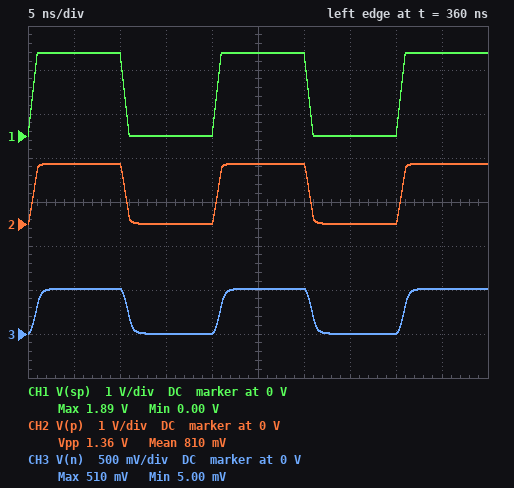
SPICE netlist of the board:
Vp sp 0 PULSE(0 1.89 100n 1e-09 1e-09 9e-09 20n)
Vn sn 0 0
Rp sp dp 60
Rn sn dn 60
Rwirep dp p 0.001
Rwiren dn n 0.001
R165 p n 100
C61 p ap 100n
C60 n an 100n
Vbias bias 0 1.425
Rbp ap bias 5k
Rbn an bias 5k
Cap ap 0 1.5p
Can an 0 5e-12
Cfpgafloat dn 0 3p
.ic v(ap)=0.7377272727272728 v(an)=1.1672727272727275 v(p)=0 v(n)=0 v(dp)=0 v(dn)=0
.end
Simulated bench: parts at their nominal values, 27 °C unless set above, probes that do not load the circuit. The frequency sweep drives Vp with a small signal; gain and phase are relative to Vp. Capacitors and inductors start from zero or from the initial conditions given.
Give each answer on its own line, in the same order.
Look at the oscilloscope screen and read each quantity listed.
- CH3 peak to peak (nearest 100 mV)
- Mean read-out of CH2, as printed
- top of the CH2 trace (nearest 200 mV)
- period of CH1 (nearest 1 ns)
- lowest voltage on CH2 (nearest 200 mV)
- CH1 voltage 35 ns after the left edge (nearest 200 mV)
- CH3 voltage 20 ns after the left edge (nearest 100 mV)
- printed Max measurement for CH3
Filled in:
500 mV
810 mV
1.4 V
20 ns
0 V
0 V
0 V
510 mV
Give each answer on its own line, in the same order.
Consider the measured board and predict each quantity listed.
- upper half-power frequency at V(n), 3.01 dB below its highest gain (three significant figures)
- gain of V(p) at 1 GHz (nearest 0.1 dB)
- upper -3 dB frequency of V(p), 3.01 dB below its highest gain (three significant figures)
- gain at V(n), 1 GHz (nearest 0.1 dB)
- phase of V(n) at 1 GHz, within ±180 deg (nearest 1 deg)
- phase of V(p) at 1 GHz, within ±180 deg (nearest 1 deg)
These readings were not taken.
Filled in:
437 MHz
-4.6 dB
1.92 GHz
-19.7 dB
-85 deg
-23 deg
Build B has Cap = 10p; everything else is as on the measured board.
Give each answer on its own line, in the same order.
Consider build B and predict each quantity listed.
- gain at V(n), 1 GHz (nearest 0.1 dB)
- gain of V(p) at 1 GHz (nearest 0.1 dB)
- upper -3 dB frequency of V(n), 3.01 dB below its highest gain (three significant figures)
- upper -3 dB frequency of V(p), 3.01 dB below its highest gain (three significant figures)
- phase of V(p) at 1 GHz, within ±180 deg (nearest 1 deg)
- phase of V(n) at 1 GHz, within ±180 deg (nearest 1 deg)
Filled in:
-27.5 dB
-12.4 dB
255 MHz
325 MHz
-68 deg
-130 deg
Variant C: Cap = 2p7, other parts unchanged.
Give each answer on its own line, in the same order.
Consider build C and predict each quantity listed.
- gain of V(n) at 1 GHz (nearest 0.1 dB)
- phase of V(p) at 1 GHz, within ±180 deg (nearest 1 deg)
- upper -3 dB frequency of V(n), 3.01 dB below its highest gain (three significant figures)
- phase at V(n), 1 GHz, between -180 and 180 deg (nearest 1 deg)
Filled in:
-20.8 dB
-35 deg
408 MHz
-97 deg
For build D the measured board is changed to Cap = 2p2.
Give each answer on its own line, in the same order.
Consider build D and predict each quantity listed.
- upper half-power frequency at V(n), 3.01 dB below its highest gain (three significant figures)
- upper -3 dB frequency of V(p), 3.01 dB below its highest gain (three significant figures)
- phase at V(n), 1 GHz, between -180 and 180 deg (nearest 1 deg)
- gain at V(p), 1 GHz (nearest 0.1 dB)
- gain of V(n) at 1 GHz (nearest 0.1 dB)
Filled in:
421 MHz
1.31 GHz
-92 deg
-5.2 dB
-20.3 dB
